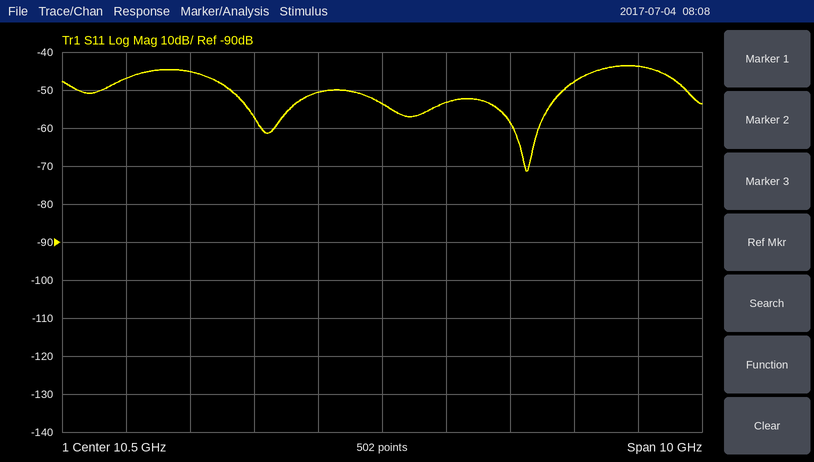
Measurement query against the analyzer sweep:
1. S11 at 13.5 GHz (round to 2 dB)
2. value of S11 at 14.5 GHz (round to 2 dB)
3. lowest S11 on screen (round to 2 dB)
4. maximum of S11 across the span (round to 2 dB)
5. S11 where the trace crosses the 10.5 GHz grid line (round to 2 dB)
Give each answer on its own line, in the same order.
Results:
-48 dB
-44 dB
-72 dB
-44 dB
-54 dB
